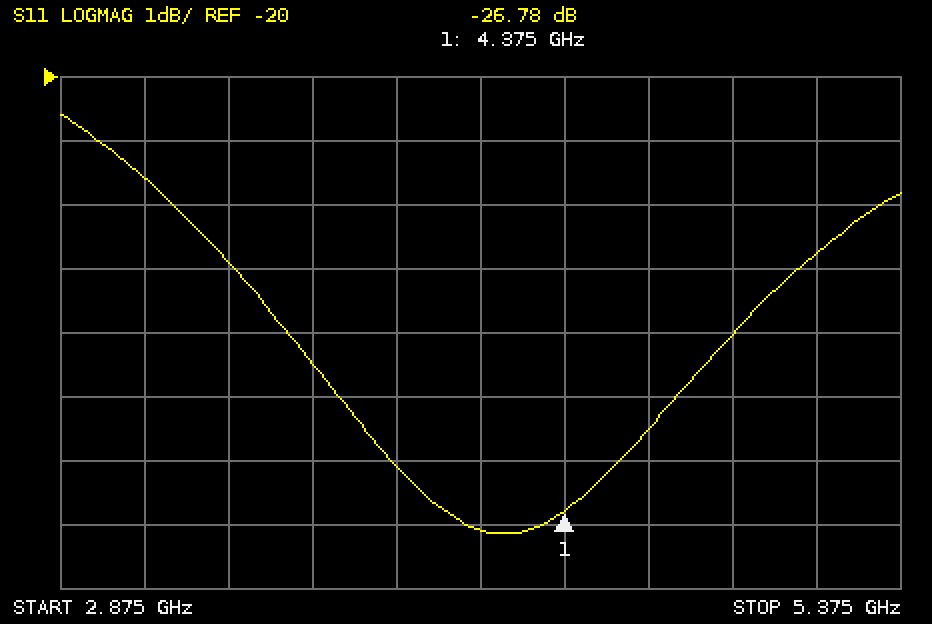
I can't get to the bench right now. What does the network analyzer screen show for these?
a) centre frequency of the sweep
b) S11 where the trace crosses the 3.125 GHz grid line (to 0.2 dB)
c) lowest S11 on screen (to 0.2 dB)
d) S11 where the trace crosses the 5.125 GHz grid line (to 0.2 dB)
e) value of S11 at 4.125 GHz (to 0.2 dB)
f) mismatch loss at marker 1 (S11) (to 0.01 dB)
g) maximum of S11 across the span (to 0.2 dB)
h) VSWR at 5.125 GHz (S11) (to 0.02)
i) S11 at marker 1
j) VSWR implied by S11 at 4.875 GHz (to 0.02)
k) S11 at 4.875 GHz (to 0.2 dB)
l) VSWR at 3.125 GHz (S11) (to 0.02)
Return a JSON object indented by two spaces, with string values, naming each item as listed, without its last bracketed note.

{
  "centre frequency of the sweep": "4.125 GHz",
  "S11 where the trace crosses the 3.125 GHz grid line": "-21.6 dB",
  "lowest S11 on screen": "-27.2 dB",
  "S11 where the trace crosses the 5.125 GHz grid line": "-22.8 dB",
  "value of S11 at 4.125 GHz": "-27.0 dB",
  "mismatch loss at marker 1 (S11)": "0.01 dB",
  "maximum of S11 across the span": "-20.6 dB",
  "VSWR at 5.125 GHz (S11)": "1.16",
  "S11 at marker 1": "-26.78 dB",
  "VSWR implied by S11 at 4.875 GHz": "1.14",
  "S11 at 4.875 GHz": "-24.0 dB",
  "VSWR at 3.125 GHz (S11)": "1.18"
}
